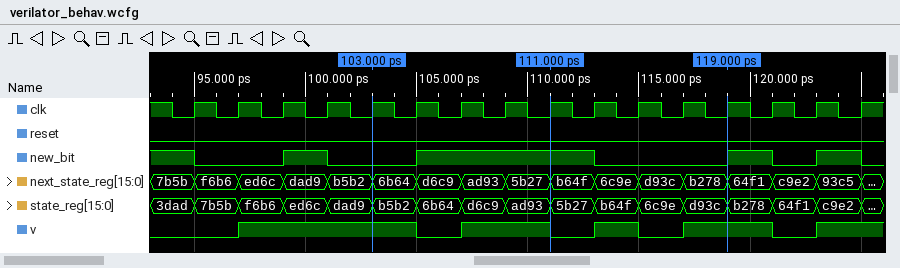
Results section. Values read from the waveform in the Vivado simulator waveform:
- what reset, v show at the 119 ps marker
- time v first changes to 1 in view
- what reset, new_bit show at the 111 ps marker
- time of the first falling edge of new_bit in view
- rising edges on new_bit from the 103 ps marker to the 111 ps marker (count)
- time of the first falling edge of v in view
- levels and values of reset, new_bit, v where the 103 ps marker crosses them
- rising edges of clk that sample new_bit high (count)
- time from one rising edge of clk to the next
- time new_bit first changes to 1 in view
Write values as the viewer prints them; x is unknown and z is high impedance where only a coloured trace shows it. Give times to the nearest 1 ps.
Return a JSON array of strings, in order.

["reset=0, v=1", "97 ps", "reset=0, new_bit=1", "95 ps", "1", "105 ps", "reset=0, new_bit=0, v=1", "8", "2 ps", "99 ps"]
